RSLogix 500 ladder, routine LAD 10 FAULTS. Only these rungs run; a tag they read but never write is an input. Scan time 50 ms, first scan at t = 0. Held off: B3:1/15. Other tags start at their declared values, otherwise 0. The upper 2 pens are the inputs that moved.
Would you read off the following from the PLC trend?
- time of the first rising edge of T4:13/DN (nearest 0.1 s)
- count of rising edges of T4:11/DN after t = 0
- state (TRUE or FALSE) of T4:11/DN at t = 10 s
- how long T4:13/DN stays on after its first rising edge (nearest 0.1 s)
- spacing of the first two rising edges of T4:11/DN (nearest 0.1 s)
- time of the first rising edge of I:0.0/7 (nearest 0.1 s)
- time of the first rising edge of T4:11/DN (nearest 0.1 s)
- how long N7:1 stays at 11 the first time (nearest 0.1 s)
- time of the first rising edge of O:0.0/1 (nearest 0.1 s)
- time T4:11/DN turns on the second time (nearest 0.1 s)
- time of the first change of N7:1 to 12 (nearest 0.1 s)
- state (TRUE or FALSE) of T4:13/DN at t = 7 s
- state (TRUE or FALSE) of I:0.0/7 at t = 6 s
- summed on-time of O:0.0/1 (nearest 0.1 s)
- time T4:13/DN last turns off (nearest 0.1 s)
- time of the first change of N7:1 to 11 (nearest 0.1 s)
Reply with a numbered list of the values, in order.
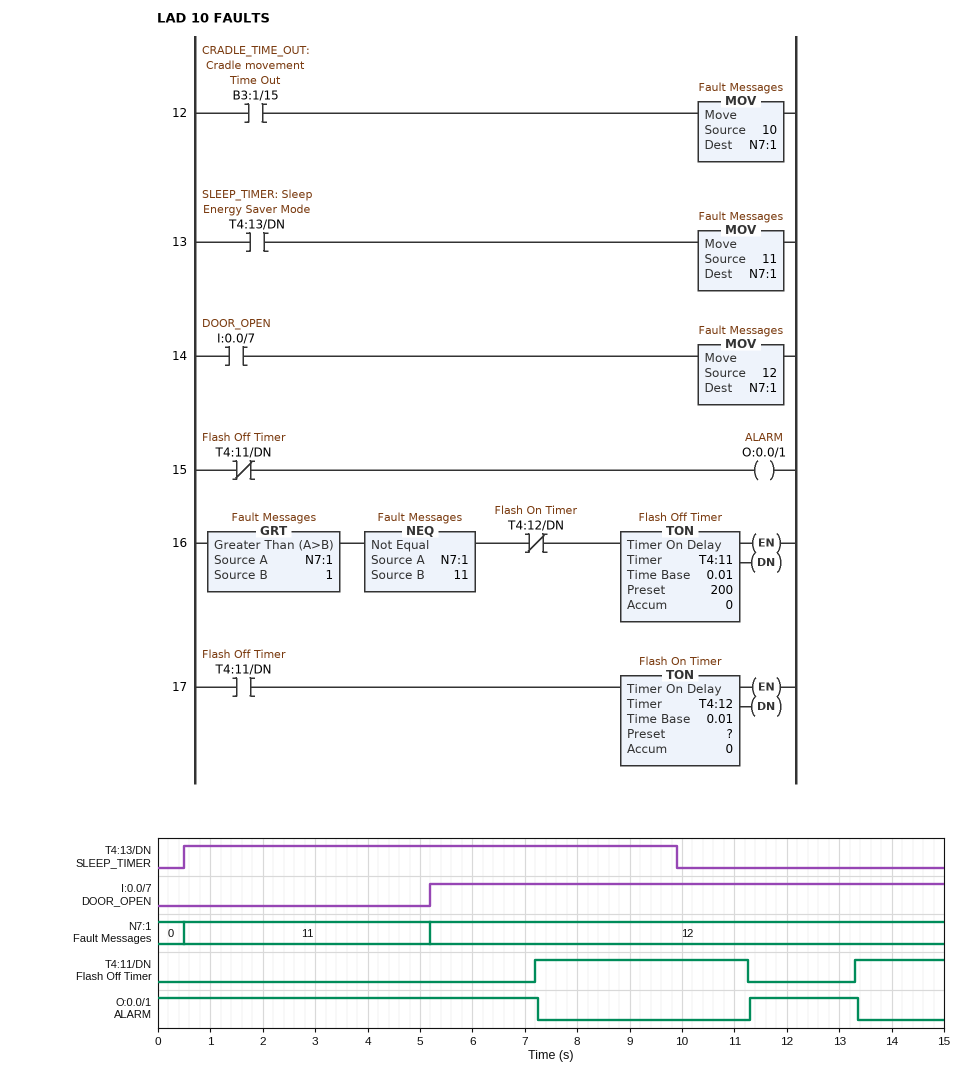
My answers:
1. 0.5 s
2. 2
3. TRUE
4. 9.4 s
5. 6.1 s
6. 5.2 s
7. 7.2 s
8. 4.7 s
9. 11.3 s
10. 13.3 s
11. 5.2 s
12. TRUE
13. TRUE
14. 9.3 s
15. 9.9 s
16. 0.5 s
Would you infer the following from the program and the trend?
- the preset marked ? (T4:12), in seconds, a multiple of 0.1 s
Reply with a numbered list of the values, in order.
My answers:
1. 4.0 s
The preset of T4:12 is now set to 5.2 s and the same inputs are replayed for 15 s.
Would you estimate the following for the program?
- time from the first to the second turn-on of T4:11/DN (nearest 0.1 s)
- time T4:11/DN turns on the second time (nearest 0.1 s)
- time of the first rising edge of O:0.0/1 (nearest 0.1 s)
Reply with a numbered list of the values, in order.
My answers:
1. 7.3 s
2. 14.5 s
3. 12.5 s
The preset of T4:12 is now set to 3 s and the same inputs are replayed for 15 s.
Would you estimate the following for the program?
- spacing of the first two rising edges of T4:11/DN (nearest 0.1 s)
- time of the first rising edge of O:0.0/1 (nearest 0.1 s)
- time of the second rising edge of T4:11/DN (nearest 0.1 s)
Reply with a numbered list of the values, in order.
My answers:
1. 5.1 s
2. 10.3 s
3. 12.3 s
